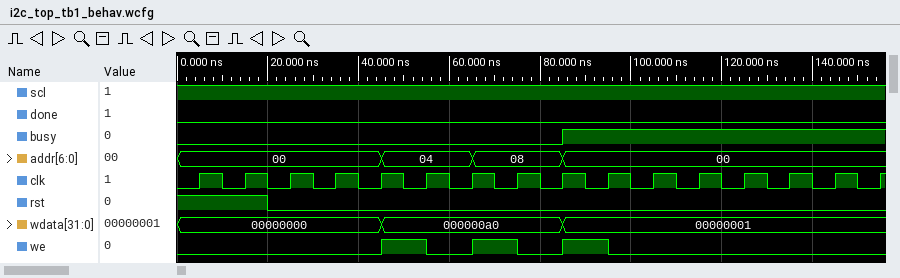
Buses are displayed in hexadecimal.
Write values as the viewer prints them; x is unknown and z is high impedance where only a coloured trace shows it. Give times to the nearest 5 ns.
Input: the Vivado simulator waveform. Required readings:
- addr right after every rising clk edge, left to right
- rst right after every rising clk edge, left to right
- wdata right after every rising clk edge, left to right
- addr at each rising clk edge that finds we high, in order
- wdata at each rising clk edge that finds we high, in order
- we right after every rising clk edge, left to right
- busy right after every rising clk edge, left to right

00, 00, 00, 00, 04, 04, 08, 08, 00, 00, 00, 00, 00, 00, 00, 00
1 1 0 0 0 0 0 0 0 0 0 0 0 0 0 0
00000000, 00000000, 00000000, 00000000, 000000a0, 000000a0, 000000a0, 000000a0, 00000001, 00000001, 00000001, 00000001, 00000001, 00000001, 00000001, 00000001
04, 08, 00
000000a0, 000000a0, 00000001
0 0 0 0 1 0 1 0 1 0 0 0 0 0 0 0
0 0 0 0 0 0 0 0 1 1 1 1 1 1 1 1
